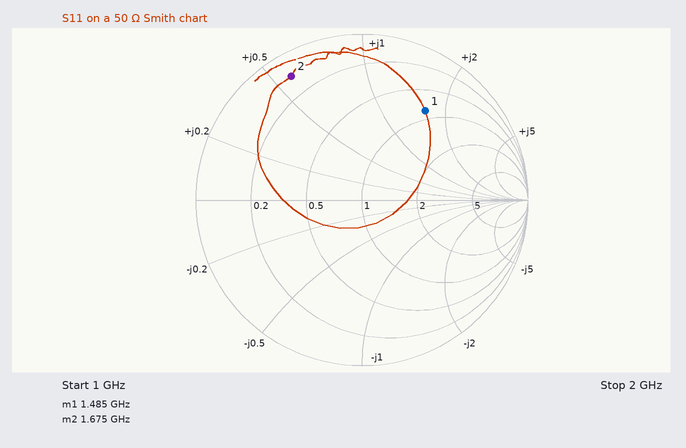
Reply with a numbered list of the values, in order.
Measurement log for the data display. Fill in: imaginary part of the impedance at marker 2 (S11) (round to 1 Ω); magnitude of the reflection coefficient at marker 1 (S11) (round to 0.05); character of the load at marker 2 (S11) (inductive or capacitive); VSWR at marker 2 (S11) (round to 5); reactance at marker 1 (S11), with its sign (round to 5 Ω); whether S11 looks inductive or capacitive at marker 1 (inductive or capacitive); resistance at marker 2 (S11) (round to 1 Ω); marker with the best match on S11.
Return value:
1. +29 Ω
2. 0.65
3. inductive
4. 15
5. +80 Ω
6. inductive
7. 5 Ω
8. marker 1
